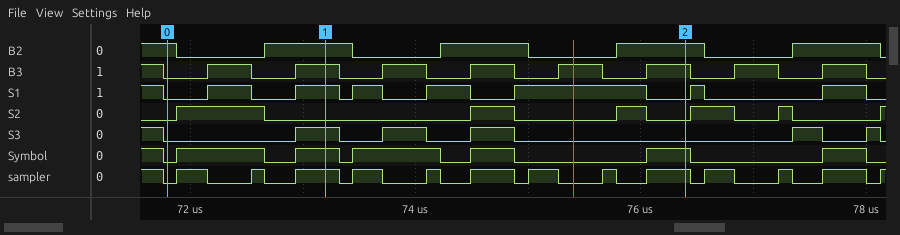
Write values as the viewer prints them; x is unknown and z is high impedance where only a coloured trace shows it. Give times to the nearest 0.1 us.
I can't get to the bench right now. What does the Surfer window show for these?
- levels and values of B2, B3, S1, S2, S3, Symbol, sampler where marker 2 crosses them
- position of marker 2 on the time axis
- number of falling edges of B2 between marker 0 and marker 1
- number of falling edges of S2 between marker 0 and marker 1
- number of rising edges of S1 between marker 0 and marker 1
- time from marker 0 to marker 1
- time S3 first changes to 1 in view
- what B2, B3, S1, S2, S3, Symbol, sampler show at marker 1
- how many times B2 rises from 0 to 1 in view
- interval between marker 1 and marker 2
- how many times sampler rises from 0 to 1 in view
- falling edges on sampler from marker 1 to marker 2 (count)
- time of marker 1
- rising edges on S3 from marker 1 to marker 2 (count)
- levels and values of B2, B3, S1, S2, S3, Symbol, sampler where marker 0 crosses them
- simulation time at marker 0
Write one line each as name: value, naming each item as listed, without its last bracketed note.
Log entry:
levels and values of B2, B3, S1, S2, S3, Symbol, sampler where marker 2 crosses them: B2=1, B3=1, S1=0, S2=0, S3=0, Symbol=1, sampler=1
position of marker 2 on the time axis: 76.4 us
number of falling edges of B2 between marker 0 and marker 1: 1
number of falling edges of S2 between marker 0 and marker 1: 1
number of rising edges of S1 between marker 0 and marker 1: 2
time from marker 0 to marker 1: 1.4 us
time S3 first changes to 1 in view: 72.9 us
what B2, B3, S1, S2, S3, Symbol, sampler show at marker 1: B2=1, B3=1, S1=1, S2=0, S3=1, Symbol=1, sampler=1
how many times B2 rises from 0 to 1 in view: 4
interval between marker 1 and marker 2: 3.2 us
how many times sampler rises from 0 to 1 in view: 13
falling edges on sampler from marker 1 to marker 2: 6
time of marker 1: 73.2 us
rising edges on S3 from marker 1 to marker 2: 2
levels and values of B2, B3, S1, S2, S3, Symbol, sampler where marker 0 crosses them: B2=1, B3=0, S1=0, S2=0, S3=0, Symbol=0, sampler=0
simulation time at marker 0: 71.8 us
